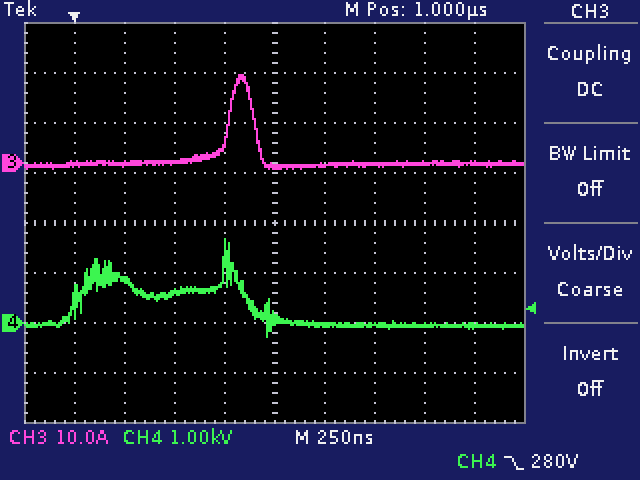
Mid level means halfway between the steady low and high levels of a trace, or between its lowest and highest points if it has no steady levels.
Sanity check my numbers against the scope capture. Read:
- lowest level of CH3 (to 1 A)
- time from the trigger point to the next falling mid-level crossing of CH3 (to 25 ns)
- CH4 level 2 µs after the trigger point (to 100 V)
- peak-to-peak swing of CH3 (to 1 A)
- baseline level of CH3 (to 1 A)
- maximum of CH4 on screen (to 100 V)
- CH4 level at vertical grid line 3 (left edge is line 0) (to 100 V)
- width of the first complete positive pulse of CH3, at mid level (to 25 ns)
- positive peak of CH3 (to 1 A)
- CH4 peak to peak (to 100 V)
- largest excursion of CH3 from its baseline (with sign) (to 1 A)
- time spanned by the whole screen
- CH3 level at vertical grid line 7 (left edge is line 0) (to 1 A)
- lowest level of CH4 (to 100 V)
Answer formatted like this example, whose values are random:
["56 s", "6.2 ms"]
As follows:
["-1 A", "900 ns", "-100 V", "19 A", "0 A", "1.7 kV", "600 V", "125 ns", "18 A", "2.0 kV", "+18 A", "2.5 µs", "0 A", "-300 V"]
